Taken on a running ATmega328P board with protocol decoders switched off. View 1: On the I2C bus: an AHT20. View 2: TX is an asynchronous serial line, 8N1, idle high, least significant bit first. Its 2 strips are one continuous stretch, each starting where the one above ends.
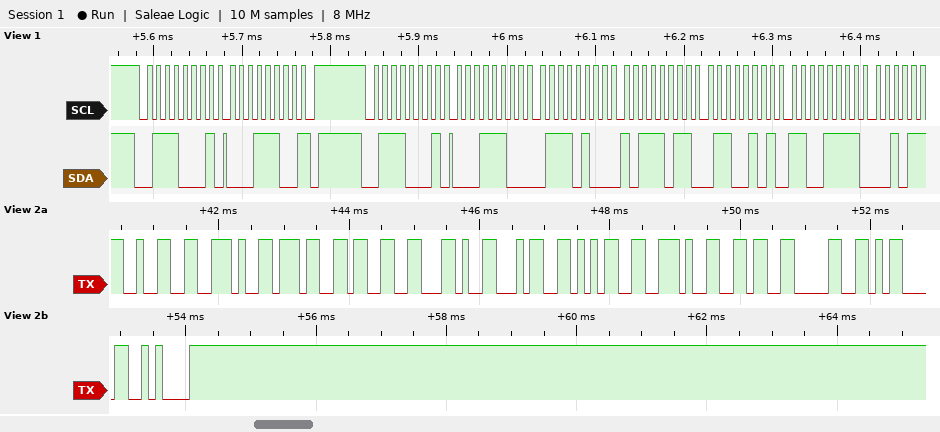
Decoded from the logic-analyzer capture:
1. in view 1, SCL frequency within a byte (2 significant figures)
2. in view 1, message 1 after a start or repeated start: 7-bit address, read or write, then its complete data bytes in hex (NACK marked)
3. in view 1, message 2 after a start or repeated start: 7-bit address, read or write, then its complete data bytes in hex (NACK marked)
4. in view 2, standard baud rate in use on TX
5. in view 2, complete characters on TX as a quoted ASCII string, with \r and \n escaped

100 kHz
0x38 read: 1C NACK
0x38 read: 1C 74 BB 65 CF
9600 baud
"2.73,45.60\r\n"
